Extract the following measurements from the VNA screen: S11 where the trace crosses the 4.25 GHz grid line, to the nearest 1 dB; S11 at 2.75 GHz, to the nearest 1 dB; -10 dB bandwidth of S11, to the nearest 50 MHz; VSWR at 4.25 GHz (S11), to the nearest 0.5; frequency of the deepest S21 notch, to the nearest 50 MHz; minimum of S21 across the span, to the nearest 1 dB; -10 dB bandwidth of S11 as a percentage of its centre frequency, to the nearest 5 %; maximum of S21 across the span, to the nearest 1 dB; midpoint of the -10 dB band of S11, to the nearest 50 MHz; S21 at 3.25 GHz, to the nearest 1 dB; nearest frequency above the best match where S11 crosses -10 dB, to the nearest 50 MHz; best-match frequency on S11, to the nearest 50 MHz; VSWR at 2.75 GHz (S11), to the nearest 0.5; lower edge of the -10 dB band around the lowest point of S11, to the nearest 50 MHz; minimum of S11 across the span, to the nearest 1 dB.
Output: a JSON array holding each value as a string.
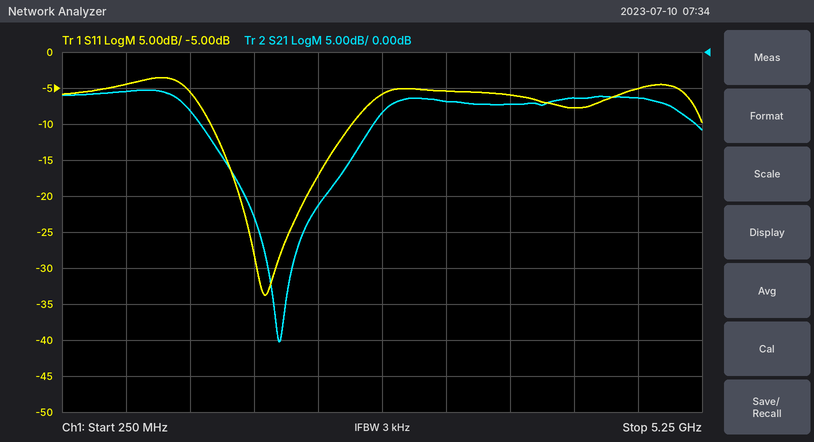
["-8 dB", "-6 dB", "1.10 GHz", "2.5", "1.95 GHz", "-40 dB", "55 %", "-5 dB", "1.95 GHz", "-7 dB", "2.50 GHz", "1.85 GHz", "3.0", "1.40 GHz", "-34 dB"]
